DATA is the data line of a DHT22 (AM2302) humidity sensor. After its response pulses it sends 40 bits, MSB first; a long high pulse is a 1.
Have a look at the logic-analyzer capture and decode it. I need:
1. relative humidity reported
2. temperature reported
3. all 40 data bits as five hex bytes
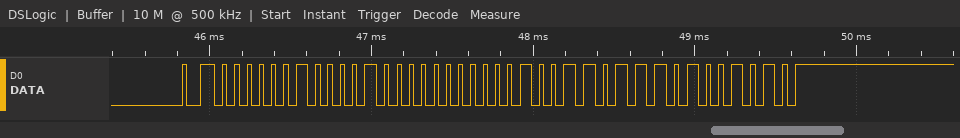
52.8 %
31.1 °C
02 10 01 37 4A
